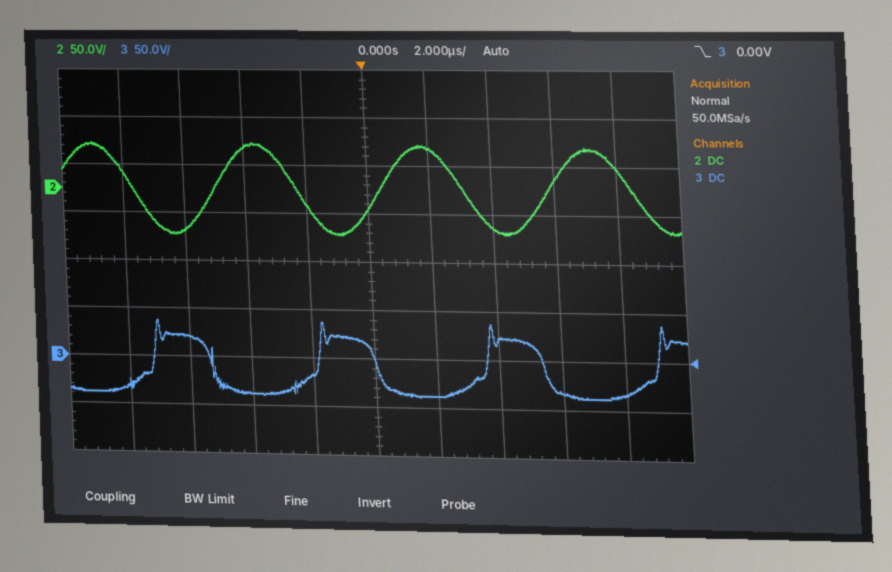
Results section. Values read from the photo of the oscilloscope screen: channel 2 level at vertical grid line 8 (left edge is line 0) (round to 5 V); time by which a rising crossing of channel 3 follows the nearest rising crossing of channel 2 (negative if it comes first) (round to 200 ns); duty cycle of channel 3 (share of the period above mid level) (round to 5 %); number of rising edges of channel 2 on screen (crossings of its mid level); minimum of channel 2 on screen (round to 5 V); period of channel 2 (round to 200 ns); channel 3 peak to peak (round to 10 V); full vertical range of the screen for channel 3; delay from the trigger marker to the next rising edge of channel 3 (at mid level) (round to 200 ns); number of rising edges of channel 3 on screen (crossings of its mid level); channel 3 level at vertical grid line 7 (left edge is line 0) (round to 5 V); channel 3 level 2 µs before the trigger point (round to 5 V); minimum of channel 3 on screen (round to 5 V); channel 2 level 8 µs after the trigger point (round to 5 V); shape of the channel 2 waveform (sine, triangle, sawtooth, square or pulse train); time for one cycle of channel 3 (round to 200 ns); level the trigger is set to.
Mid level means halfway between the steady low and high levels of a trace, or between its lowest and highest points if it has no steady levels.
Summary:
10 V
-2.2 µs
35 %
3
-45 V
5.4 µs
80 V
400 V
3.6 µs
4
20 V
-15 V
-40 V
25 V
sine
5.4 µs
0.00 V
